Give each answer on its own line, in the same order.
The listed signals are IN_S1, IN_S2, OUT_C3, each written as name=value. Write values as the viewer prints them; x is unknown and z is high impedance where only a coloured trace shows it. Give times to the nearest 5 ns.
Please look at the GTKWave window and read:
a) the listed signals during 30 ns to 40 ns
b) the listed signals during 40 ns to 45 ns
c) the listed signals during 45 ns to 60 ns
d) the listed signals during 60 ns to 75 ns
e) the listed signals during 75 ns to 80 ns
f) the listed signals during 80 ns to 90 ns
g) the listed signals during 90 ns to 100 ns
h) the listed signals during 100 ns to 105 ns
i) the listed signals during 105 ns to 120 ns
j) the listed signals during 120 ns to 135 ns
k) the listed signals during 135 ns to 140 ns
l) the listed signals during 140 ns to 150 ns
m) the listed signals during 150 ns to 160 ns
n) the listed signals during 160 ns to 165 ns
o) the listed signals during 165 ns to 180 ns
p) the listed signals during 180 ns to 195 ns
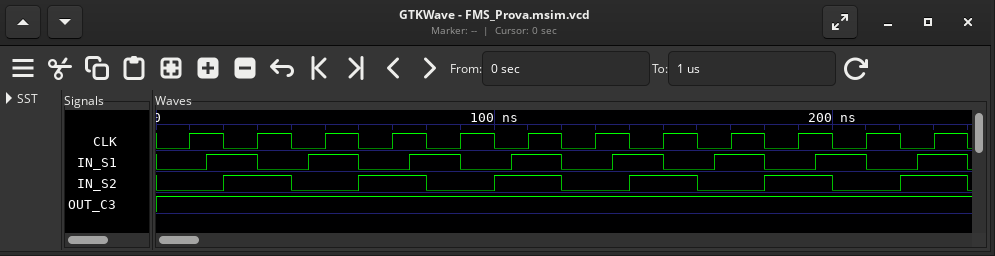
IN_S1=0, IN_S2=1, OUT_C3=1
IN_S1=0, IN_S2=0, OUT_C3=1
IN_S1=1, IN_S2=0, OUT_C3=1
IN_S1=0, IN_S2=1, OUT_C3=1
IN_S1=1, IN_S2=1, OUT_C3=1
IN_S1=1, IN_S2=0, OUT_C3=1
IN_S1=0, IN_S2=0, OUT_C3=1
IN_S1=0, IN_S2=1, OUT_C3=1
IN_S1=1, IN_S2=1, OUT_C3=1
IN_S1=0, IN_S2=0, OUT_C3=1
IN_S1=1, IN_S2=0, OUT_C3=1
IN_S1=1, IN_S2=1, OUT_C3=1
IN_S1=0, IN_S2=1, OUT_C3=1
IN_S1=0, IN_S2=0, OUT_C3=1
IN_S1=1, IN_S2=0, OUT_C3=1
IN_S1=0, IN_S2=1, OUT_C3=1
